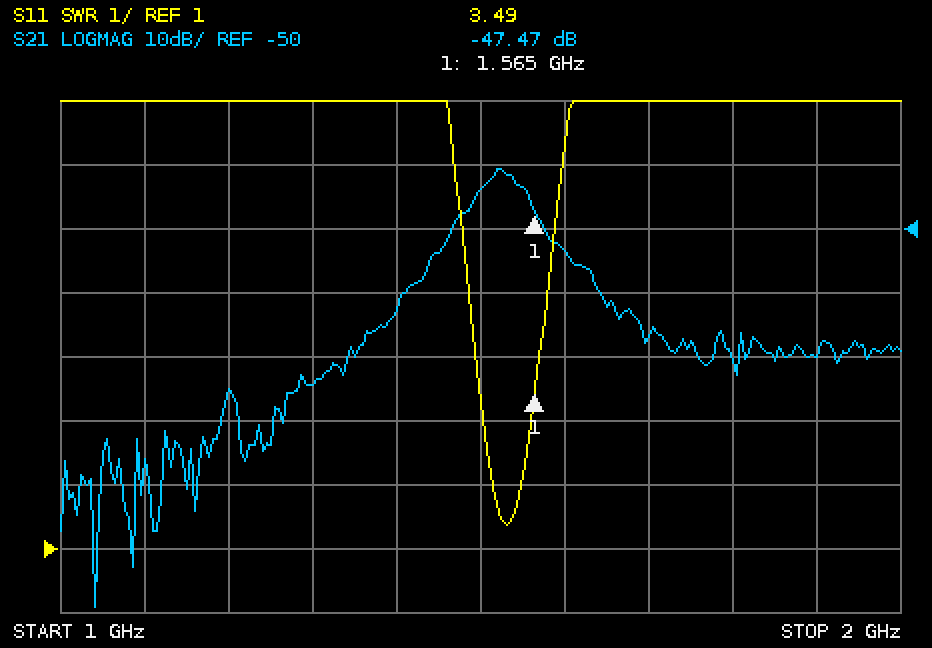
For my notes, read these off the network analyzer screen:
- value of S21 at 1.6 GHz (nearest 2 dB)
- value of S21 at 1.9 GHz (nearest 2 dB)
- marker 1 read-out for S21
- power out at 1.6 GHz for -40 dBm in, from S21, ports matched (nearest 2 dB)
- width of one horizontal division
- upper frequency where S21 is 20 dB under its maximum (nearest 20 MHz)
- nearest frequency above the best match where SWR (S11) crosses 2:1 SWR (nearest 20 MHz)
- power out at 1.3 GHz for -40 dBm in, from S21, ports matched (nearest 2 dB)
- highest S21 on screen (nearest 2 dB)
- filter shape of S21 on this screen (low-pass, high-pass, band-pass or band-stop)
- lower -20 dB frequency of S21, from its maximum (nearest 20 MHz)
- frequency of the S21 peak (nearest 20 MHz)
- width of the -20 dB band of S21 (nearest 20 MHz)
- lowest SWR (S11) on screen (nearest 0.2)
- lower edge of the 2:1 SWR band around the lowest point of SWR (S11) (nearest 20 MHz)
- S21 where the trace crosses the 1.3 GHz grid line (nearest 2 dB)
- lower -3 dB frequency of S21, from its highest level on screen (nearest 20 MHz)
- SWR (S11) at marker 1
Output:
-54 dB
-70 dB
-47.47 dB
-94 dBm
100 MHz
1.64 GHz
1.54 GHz
-114 dBm
-40 dB
band-pass
1.40 GHz
1.52 GHz
240 MHz
1.4
1.52 GHz
-74 dB
1.50 GHz
3.49
